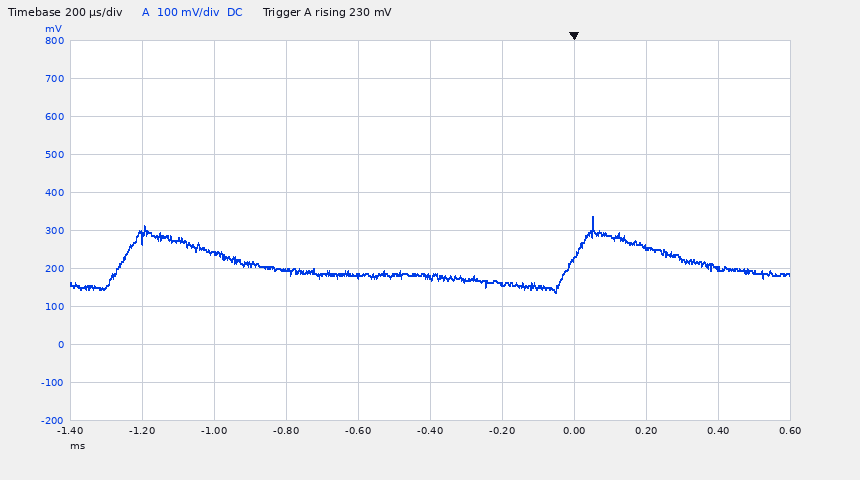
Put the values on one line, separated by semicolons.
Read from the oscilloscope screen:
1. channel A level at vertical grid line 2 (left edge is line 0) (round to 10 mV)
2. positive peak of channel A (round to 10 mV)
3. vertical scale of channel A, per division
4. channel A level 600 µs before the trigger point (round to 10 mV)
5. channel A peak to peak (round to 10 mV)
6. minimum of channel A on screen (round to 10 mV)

240 mV; 340 mV; 100 mV; 180 mV; 200 mV; 140 mV
